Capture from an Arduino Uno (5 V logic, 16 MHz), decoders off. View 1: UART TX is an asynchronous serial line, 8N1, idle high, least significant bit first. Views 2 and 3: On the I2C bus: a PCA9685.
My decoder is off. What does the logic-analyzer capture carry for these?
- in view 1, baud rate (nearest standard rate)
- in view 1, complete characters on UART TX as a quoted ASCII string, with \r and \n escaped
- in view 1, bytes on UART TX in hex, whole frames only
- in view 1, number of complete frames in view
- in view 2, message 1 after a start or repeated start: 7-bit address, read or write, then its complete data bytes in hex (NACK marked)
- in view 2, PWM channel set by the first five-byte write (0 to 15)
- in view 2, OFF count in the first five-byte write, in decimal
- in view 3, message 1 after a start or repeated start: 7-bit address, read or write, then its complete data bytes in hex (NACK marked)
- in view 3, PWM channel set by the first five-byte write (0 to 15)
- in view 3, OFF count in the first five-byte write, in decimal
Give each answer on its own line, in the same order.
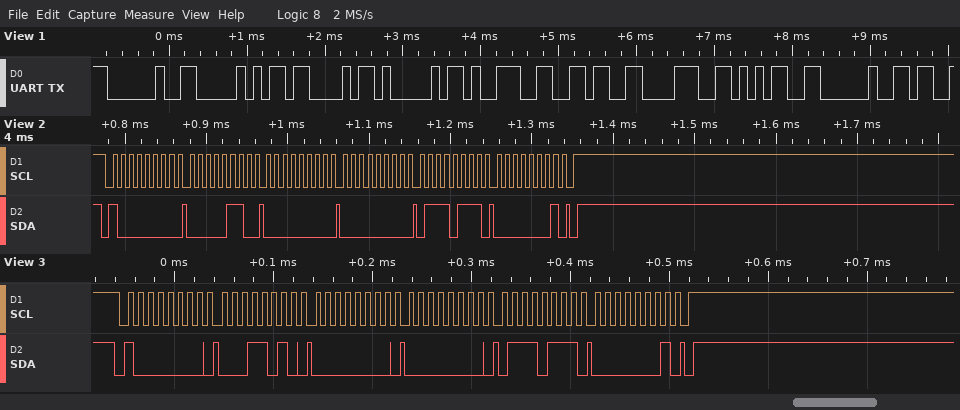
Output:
9600 baud
" PCA9685 "
20 50 43 41 39 36 38 35 20
9
0x40 write: 06 00 00 77 01
0
375
0x40 write: 1A 00 00 77 01
5
375
